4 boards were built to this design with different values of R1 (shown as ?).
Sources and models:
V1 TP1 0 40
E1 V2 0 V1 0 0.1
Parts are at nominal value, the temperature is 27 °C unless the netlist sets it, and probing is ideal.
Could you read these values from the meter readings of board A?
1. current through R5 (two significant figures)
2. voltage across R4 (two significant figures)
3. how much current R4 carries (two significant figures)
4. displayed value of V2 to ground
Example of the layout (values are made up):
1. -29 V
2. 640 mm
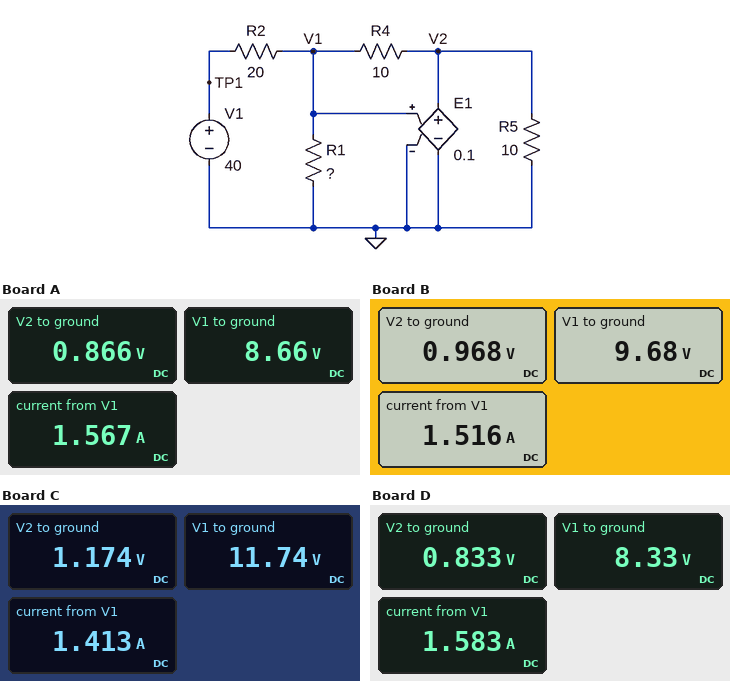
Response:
1. 87 mA
2. 7.8 V
3. 780 mA
4. 0.866 V
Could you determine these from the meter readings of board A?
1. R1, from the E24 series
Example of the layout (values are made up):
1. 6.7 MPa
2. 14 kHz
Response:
1. 11 Ω
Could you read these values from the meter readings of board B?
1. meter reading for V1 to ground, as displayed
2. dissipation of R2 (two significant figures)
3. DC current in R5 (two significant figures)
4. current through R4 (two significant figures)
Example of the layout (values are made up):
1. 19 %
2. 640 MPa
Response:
1. 9.68 V
2. 46 W
3. 97 mA
4. 870 mA
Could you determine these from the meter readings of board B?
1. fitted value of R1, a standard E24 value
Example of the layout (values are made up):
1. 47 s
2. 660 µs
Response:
1. 15 Ω
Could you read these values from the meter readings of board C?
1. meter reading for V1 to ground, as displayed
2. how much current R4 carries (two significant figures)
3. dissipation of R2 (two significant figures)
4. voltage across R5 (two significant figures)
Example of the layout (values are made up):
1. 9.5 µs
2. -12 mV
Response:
1. 11.74 V
2. 1.1 A
3. 40 W
4. 1.2 V
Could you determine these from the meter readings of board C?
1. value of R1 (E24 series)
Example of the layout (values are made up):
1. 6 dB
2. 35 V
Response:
1. 33 Ω
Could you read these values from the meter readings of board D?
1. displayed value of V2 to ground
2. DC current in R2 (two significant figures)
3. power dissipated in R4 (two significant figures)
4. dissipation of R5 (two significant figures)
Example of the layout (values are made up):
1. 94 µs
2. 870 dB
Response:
1. 0.833 V
2. 1.6 A
3. 5.6 W
4. 69 mW
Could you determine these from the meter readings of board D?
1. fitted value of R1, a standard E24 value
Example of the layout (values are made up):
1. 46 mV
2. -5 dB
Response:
1. 10 Ω
